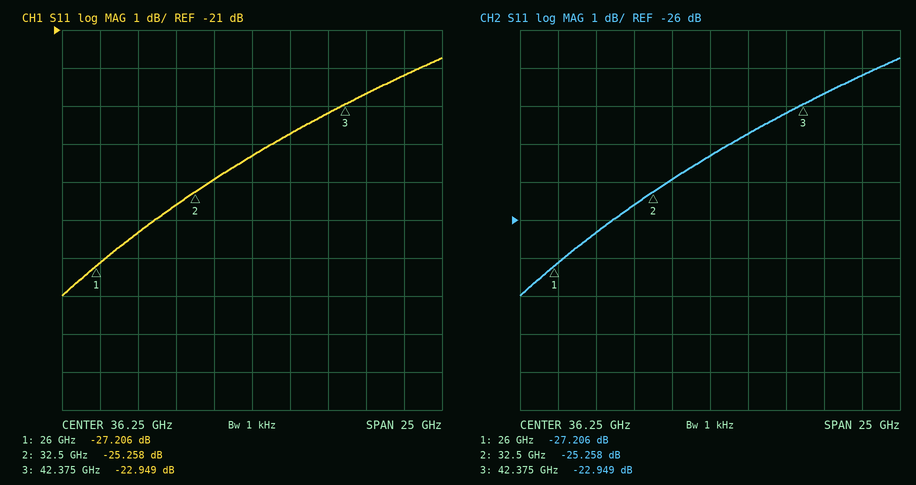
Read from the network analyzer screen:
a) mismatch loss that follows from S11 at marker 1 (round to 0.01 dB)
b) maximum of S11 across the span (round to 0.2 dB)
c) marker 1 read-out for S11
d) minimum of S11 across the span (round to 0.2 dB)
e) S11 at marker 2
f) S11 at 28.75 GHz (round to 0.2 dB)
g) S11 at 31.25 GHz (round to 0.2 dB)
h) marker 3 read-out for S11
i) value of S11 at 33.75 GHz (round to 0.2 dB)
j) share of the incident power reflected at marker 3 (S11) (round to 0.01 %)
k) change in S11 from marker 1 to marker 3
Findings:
0.01 dB
-21.8 dB
-27.206 dB
-28.0 dB
-25.258 dB
-26.4 dB
-25.6 dB
-22.949 dB
-25.0 dB
0.51 %
4.257 dB
